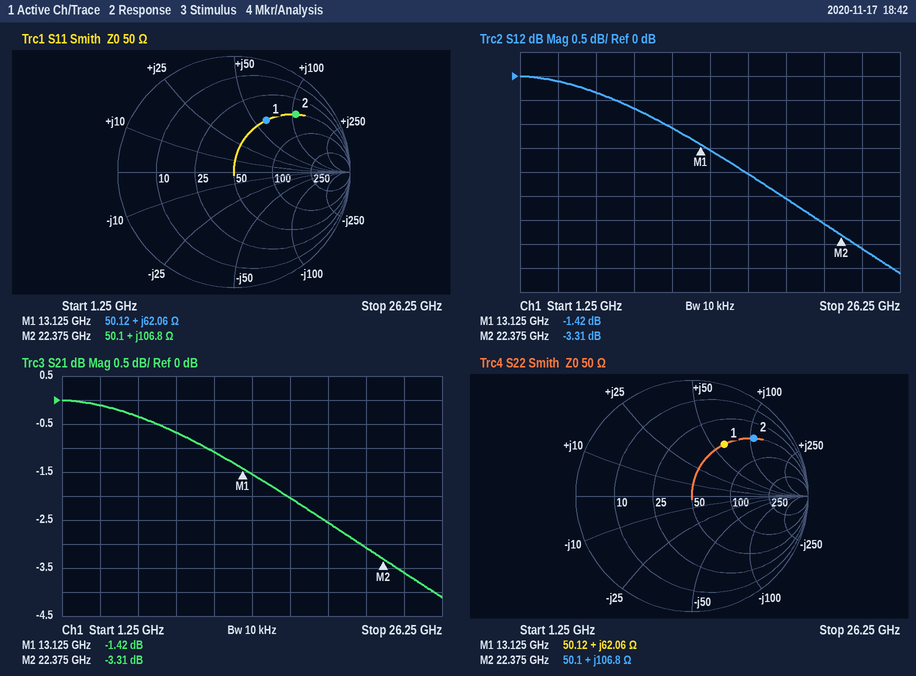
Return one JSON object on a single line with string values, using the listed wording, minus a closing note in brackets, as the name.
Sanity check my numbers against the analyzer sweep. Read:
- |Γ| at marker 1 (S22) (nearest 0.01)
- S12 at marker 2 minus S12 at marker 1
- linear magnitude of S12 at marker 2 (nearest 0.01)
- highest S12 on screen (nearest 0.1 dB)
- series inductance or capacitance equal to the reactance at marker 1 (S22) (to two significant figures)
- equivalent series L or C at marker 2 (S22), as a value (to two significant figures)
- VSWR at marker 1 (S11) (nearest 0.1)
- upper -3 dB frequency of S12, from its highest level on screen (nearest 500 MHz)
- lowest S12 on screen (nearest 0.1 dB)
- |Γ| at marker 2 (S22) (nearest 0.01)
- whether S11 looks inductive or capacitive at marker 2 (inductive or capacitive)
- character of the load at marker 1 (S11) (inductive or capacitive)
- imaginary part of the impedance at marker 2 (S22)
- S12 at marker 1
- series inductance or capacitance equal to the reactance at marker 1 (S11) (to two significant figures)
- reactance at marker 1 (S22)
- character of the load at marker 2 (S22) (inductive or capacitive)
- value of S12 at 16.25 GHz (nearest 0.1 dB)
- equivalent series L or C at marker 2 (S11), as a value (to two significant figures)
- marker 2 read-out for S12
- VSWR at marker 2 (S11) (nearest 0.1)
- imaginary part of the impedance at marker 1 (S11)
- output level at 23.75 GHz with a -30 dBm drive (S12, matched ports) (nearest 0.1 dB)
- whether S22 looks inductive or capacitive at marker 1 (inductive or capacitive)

{"|Γ| at marker 1 (S22)": "0.53", "S12 at marker 2 minus S12 at marker 1": "-1.89 dB", "linear magnitude of S12 at marker 2": "0.68", "highest S12 on screen": "0.0 dB", "series inductance or capacitance equal to the reactance at marker 1 (S22)": "750 pH", "equivalent series L or C at marker 2 (S22), as a value": "760 pH", "VSWR at marker 1 (S11)": "3.2", "upper -3 dB frequency of S12, from its highest level on screen": "21.0 GHz", "lowest S12 on screen": "-4.1 dB", "|Γ| at marker 2 (S22)": "0.73", "whether S11 looks inductive or capacitive at marker 2": "inductive", "character of the load at marker 1 (S11)": "inductive", "imaginary part of the impedance at marker 2": "+106.8 Ω", "S12 at marker 1": "-1.42 dB", "series inductance or capacitance equal to the reactance at marker 1 (S11)": "750 pH", "reactance at marker 1": "+62.06 Ω", "character of the load at marker 2 (S22)": "inductive", "value of S12 at 16.25 GHz": "-2.0 dB", "equivalent series L or C at marker 2 (S11), as a value": "760 pH", "marker 2 read-out for S12": "-3.31 dB", "VSWR at marker 2 (S11)": "6.4", "imaginary part of the impedance at marker 1": "+62.06 Ω", "output level at 23.75 GHz with a -30 dBm drive (S12, matched ports)": "-33.6 dBm", "whether S22 looks inductive or capacitive at marker 1": "inductive"}
